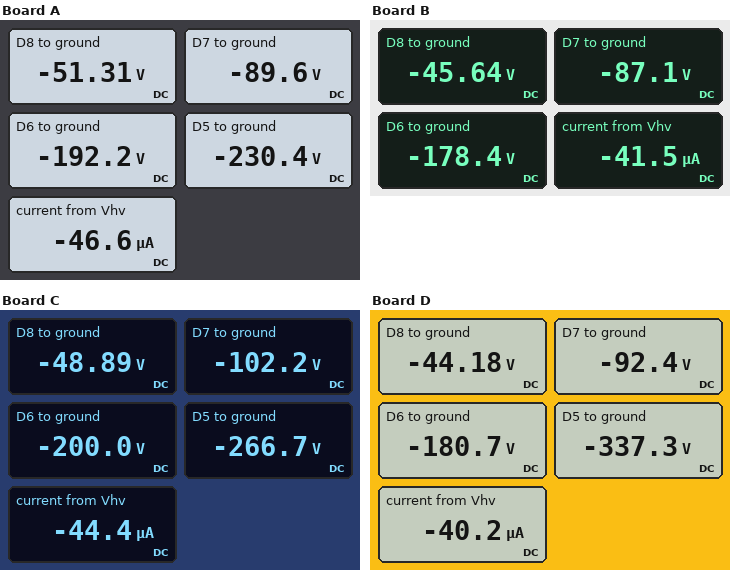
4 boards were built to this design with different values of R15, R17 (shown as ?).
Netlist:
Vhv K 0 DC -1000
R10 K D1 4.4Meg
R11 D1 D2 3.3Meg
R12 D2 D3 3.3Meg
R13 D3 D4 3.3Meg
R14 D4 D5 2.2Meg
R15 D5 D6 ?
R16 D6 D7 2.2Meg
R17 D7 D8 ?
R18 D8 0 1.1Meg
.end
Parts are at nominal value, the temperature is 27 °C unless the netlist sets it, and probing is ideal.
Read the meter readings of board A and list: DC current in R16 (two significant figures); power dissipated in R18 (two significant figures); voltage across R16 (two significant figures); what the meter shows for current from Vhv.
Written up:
47 µA
2.4 mW
100 V
-46.6 µA
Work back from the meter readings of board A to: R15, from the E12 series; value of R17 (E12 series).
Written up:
820 kΩ
820 kΩ
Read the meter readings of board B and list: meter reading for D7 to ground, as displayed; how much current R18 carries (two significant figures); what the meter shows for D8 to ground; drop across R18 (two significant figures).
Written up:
-87.1 V
41 µA
-45.64 V
46 V
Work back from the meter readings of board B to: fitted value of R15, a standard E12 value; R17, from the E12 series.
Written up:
3.3 MΩ
1 MΩ
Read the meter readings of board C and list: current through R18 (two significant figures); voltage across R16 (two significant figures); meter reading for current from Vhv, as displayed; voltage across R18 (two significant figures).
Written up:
44 µA
98 V
-44.4 µA
49 V
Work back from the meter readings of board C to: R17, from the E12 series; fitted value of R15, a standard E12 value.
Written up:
1.2 MΩ
1.5 MΩ
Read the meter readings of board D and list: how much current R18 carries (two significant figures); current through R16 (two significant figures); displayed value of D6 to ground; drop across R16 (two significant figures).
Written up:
40 µA
40 µA
-180.7 V
88 V
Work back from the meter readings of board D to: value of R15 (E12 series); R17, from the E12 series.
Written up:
3.9 MΩ
1.2 MΩ
